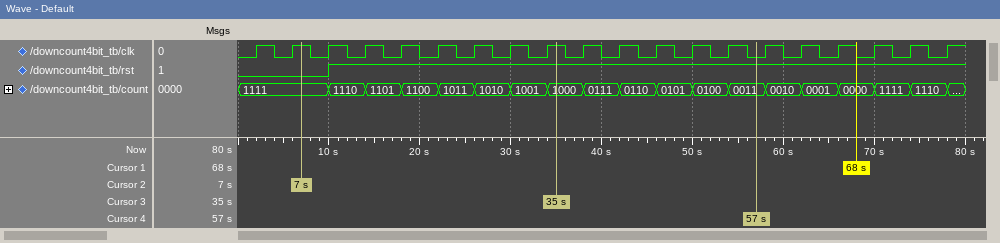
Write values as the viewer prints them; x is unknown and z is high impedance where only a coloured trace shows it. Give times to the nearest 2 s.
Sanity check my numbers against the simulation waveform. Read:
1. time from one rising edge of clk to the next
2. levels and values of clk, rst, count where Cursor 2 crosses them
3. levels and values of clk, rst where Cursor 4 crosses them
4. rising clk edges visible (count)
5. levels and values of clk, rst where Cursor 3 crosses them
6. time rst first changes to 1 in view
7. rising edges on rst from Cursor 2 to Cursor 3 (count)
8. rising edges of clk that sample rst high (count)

4 s
clk=1, rst=0, count=1111
clk=0, rst=1
20
clk=1, rst=1
10 s
1
17
